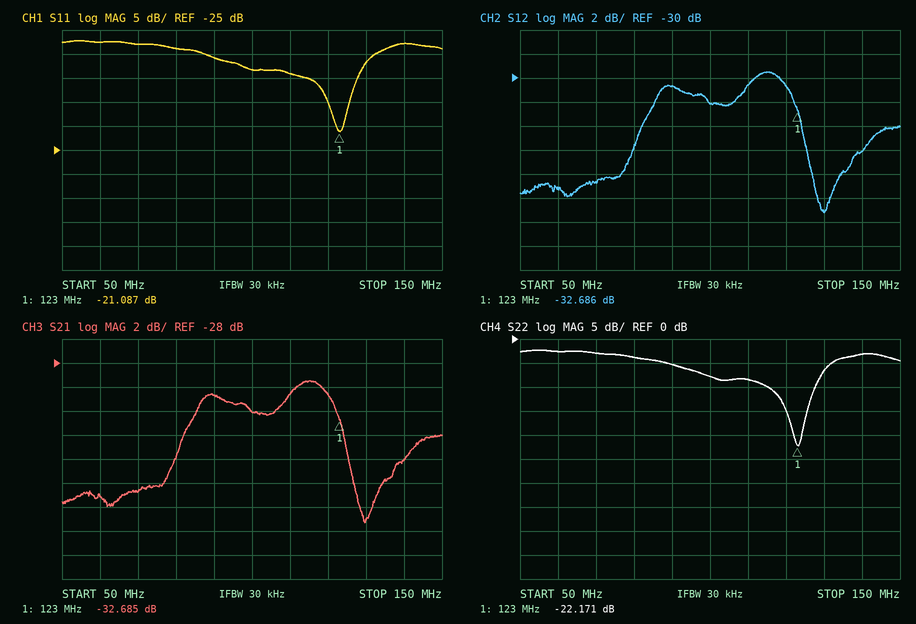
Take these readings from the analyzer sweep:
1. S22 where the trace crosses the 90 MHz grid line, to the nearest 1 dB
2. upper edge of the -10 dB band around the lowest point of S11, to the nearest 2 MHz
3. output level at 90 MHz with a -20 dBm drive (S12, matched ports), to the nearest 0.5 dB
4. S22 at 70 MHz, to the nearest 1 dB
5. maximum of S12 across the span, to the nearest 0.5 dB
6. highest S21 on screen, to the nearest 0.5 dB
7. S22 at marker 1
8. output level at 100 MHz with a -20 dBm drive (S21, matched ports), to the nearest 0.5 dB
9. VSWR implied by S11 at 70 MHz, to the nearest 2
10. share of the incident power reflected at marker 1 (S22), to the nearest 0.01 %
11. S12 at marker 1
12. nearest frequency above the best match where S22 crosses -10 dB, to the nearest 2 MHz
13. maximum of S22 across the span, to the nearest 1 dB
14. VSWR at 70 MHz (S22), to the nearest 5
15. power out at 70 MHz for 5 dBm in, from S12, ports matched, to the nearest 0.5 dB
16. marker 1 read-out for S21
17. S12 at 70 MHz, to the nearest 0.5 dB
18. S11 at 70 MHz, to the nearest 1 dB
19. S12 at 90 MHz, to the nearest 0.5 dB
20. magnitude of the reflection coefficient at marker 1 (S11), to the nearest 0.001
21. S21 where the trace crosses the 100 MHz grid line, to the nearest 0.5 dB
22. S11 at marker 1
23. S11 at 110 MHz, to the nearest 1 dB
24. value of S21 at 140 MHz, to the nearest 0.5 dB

-5 dB
128 MHz
-50.5 dBm
-3 dB
-29.5 dB
-29.5 dB
-22.171 dB
-52.0 dBm
6
0.61 %
-32.686 dB
128 MHz
-2 dB
5
-33.5 dBm
-32.685 dB
-38.5 dB
-3 dB
-30.5 dB
0.088
-32.0 dB
-21.087 dB
-9 dB
-36.0 dB
